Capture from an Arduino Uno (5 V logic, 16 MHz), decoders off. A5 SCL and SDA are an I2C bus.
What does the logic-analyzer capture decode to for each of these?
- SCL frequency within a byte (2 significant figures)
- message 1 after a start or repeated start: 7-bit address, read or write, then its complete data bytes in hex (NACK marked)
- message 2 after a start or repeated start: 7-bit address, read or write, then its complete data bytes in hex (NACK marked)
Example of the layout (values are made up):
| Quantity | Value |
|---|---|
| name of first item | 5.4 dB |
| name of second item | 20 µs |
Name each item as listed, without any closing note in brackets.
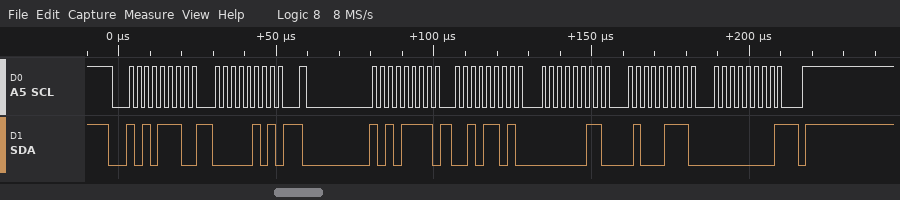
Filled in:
| Quantity | Value |
|---|---|
| SCL frequency within a byte | 400 kHz |
| message 1 after a start or repeated start: 7-bit address, read or write, then its complete data bytes in hex | 0x57 write: 05 |
| message 2 after a start or repeated start: 7-bit address, read or write, then its complete data bytes in hex | 0x57 read: 2D 03 47 00 NACK |
